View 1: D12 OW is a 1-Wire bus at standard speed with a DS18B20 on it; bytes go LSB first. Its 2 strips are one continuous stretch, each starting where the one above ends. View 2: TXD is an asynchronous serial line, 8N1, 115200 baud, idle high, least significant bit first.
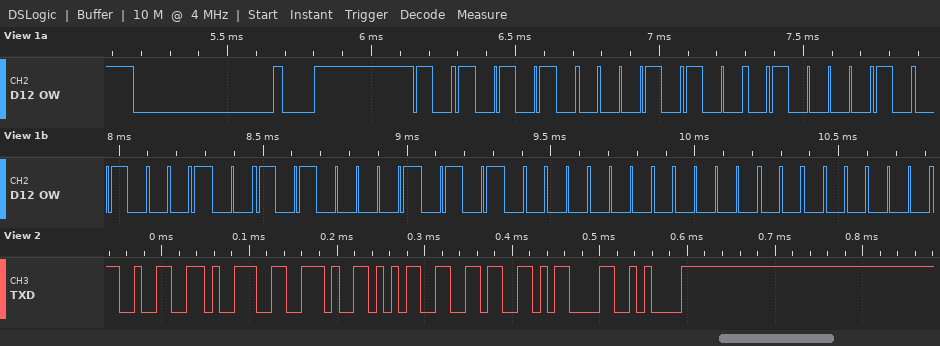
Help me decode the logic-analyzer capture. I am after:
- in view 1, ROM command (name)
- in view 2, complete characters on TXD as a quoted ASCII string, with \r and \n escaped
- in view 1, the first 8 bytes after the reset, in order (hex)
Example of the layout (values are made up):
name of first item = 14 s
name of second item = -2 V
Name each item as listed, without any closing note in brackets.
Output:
in view 1, ROM command = Match ROM
in view 2, complete characters on TXD as a quoted ASCII string, with \r and \n escaped = "29.56\r\n"
in view 1, the first 8 bytes after the reset, in order = 55 28 42 22 85 0A 00 00
